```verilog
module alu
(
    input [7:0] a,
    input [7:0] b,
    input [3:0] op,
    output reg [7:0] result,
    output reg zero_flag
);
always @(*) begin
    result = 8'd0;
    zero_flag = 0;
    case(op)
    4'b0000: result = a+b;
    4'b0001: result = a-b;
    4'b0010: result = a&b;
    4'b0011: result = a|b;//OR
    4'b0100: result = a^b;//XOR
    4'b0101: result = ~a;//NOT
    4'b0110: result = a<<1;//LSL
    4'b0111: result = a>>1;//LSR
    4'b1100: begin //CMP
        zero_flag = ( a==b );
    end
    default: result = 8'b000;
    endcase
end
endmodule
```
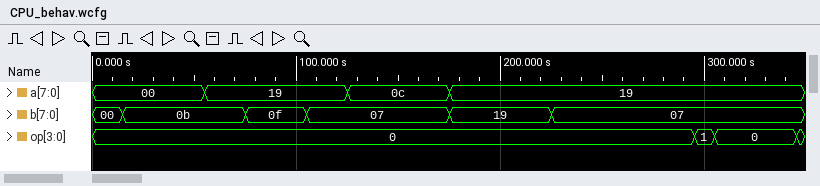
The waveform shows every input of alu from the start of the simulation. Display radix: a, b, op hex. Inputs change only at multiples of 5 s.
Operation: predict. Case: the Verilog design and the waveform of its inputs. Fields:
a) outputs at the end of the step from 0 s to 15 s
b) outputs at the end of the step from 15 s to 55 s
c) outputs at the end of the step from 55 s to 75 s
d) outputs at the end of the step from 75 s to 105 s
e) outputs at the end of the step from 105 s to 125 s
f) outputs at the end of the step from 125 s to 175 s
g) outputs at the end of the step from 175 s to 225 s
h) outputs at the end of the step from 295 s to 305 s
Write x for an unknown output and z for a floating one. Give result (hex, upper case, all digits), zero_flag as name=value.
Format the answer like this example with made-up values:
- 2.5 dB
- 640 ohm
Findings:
- result=00, zero_flag=0
- result=0B, zero_flag=0
- result=24, zero_flag=0
- result=28, zero_flag=0
- result=20, zero_flag=0
- result=13, zero_flag=0
- result=32, zero_flag=0
- result=12, zero_flag=0
